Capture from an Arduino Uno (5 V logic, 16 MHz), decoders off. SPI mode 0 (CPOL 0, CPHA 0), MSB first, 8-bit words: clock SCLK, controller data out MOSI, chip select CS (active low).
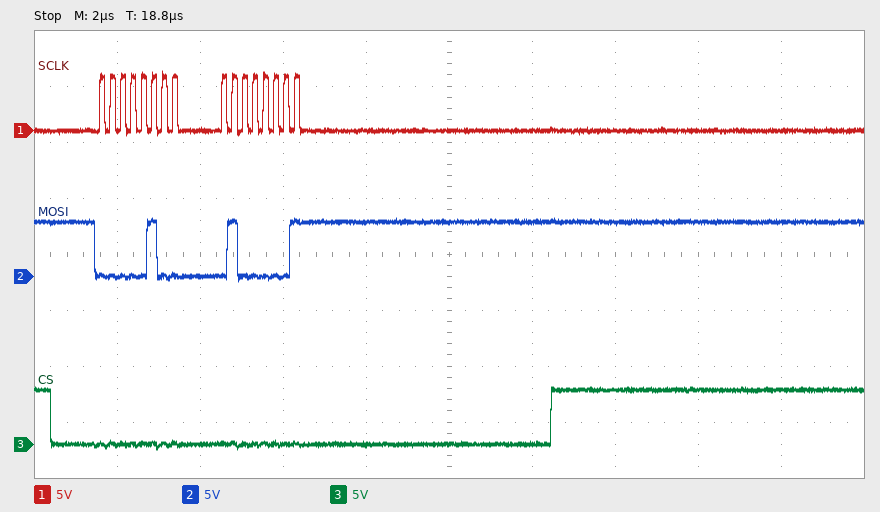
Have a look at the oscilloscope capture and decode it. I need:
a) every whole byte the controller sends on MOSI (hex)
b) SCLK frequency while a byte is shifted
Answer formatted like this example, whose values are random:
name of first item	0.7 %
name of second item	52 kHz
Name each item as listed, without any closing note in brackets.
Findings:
every whole byte the controller sends on MOSI	04 41
SCLK frequency while a byte is shifted	4 MHz
